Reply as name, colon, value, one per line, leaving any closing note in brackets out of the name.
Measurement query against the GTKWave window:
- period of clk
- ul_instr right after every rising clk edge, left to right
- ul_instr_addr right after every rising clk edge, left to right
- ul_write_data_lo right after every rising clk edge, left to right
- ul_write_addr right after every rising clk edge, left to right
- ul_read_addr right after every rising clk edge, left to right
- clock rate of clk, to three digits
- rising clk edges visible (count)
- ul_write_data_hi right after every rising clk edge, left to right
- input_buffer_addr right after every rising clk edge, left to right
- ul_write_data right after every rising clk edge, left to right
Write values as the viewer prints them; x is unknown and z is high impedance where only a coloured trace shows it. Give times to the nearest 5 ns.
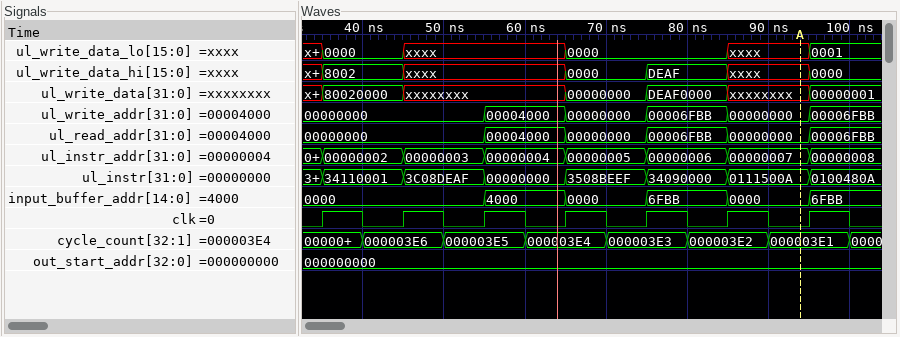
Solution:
period of clk: 10 ns
ul_instr right after every rising clk edge, left to right: 34110001, 3C08DEAF, 00000000, 3508BEEF, 34090000, 0111500A, 0100480A
ul_instr_addr right after every rising clk edge, left to right: 00000002, 00000003, 00000004, 00000005, 00000006, 00000007, 00000008
ul_write_data_lo right after every rising clk edge, left to right: 0000, xxxx, xxxx, 0000, 0000, xxxx, 0001
ul_write_addr right after every rising clk edge, left to right: 00000000, 00000000, 00004000, 00000000, 00006FBB, 00000000, 00006FBB
ul_read_addr right after every rising clk edge, left to right: 00000000, 00000000, 00004000, 00000000, 00006FBB, 00000000, 00006FBB
clock rate of clk, to three digits: 100 MHz
rising clk edges visible: 7
ul_write_data_hi right after every rising clk edge, left to right: 8002, xxxx, xxxx, 0000, DEAF, xxxx, 0000
input_buffer_addr right after every rising clk edge, left to right: 0000, 0000, 4000, 0000, 6FBB, 0000, 6FBB
ul_write_data right after every rising clk edge, left to right: 80020000, xxxxxxxx, xxxxxxxx, 00000000, DEAF0000, xxxxxxxx, 00000001
